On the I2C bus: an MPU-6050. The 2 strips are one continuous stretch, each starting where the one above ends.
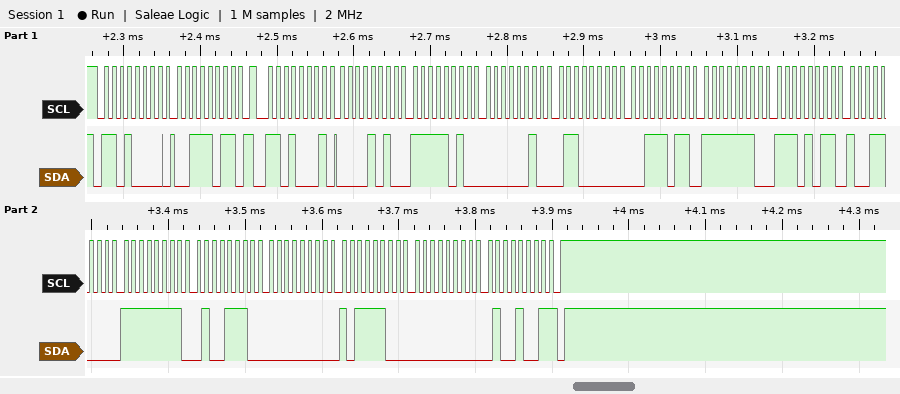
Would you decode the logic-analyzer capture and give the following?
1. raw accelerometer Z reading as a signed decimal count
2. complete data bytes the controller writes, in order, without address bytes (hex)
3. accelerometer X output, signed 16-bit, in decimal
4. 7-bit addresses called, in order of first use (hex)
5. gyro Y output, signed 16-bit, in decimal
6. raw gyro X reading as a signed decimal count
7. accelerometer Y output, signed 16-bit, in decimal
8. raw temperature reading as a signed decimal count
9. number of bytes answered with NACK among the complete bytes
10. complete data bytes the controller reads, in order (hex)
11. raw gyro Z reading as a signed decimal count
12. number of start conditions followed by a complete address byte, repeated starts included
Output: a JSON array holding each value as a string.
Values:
["15358", "3B", "2810", "0x68", "188", "-178", "608", "-5224", "1", "0A FA 02 60 3B FE EB 98 FF 4E 00 BC 00 49", "73", "2"]
